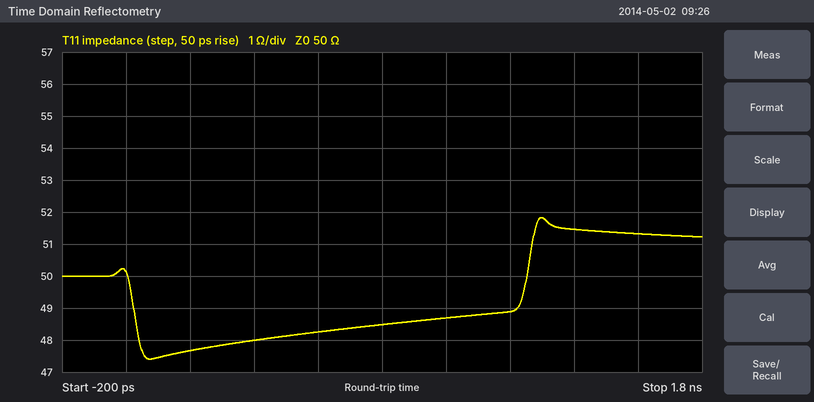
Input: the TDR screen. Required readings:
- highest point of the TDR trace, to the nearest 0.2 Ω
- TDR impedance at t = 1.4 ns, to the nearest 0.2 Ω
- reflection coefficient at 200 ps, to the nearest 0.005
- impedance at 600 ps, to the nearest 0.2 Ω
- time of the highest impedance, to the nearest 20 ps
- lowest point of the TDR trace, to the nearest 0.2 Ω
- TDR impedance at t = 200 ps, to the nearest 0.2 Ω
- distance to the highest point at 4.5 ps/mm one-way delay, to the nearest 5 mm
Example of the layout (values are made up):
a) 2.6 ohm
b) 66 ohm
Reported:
a) 51.8 Ω
b) 51.4 Ω
c) -0.025
d) 48.2 Ω
e) 1.30 ns
f) 47.4 Ω
g) 47.6 Ω
h) 145 mm
